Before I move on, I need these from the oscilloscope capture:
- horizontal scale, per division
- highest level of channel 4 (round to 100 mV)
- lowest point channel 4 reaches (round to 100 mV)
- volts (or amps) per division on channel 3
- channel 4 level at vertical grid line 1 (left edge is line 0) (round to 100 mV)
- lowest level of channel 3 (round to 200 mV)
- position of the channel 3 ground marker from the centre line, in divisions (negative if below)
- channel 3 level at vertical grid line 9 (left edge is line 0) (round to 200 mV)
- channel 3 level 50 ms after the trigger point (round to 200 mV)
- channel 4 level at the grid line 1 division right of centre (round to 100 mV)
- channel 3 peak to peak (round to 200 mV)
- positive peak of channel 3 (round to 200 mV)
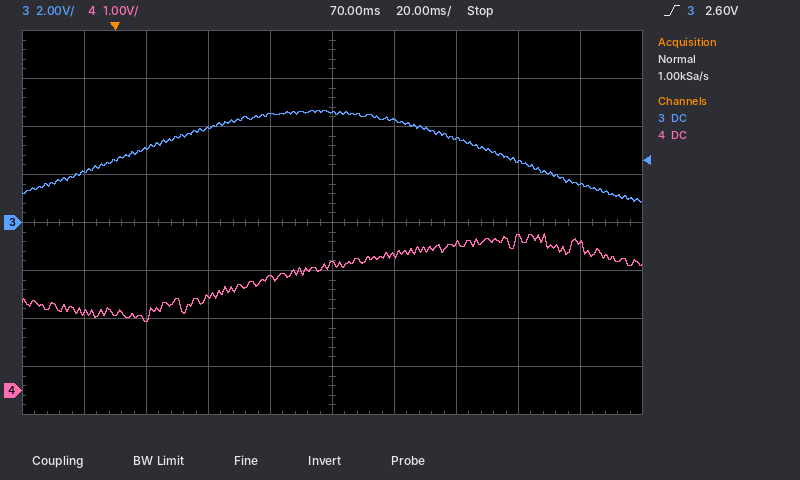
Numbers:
20 ms
3.3 V
1.4 V
2 V
1.6 V
800 mV
0.0 div
1.6 V
4.6 V
2.8 V
3.8 V
4.6 V
